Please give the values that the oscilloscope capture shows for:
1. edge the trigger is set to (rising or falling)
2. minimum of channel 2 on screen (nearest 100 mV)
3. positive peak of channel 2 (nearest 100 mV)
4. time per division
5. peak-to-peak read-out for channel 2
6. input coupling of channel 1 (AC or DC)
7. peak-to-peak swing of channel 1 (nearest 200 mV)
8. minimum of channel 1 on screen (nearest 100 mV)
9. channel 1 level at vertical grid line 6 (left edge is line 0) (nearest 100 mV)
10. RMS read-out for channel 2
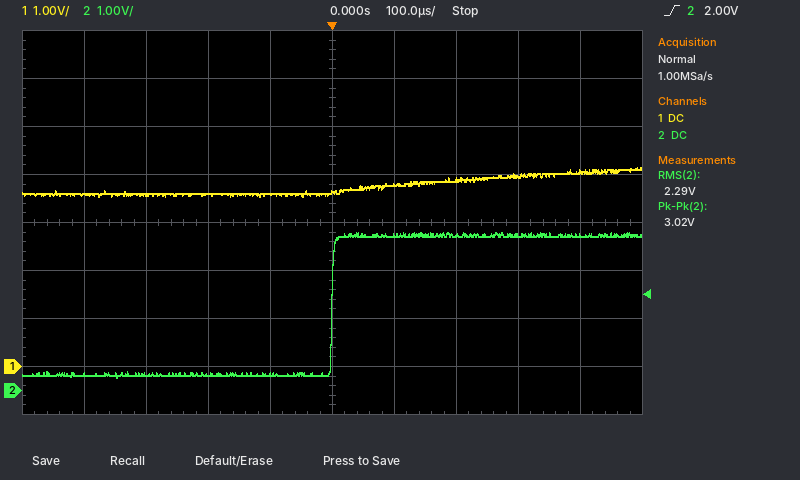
rising
300 mV
3.3 V
100 µs
3.02 V
DC
600 mV
3.5 V
3.8 V
2.29 V
